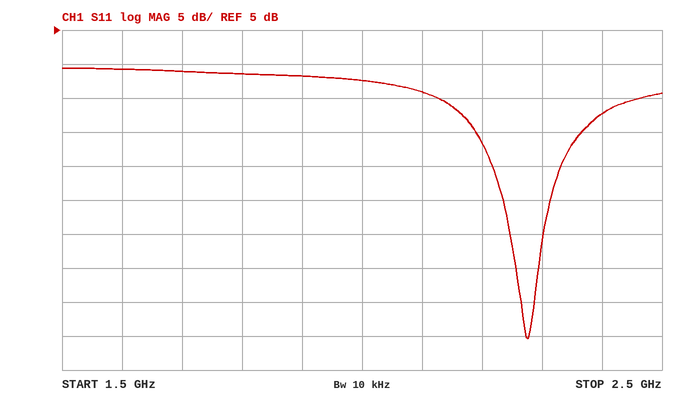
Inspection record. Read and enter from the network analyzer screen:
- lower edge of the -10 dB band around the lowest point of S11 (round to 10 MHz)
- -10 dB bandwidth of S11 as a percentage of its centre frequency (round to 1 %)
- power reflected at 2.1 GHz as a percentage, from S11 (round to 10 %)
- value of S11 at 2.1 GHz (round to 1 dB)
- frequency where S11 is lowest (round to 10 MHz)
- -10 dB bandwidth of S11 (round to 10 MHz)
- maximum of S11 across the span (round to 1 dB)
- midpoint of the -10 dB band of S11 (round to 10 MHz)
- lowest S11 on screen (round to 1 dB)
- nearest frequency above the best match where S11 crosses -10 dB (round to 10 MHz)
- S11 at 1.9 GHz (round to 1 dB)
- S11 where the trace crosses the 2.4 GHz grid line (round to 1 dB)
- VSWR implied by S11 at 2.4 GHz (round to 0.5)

2.19 GHz
8 %
40 %
-4 dB
2.28 GHz
180 MHz
-1 dB
2.28 GHz
-40 dB
2.37 GHz
-2 dB
-7 dB
2.5
